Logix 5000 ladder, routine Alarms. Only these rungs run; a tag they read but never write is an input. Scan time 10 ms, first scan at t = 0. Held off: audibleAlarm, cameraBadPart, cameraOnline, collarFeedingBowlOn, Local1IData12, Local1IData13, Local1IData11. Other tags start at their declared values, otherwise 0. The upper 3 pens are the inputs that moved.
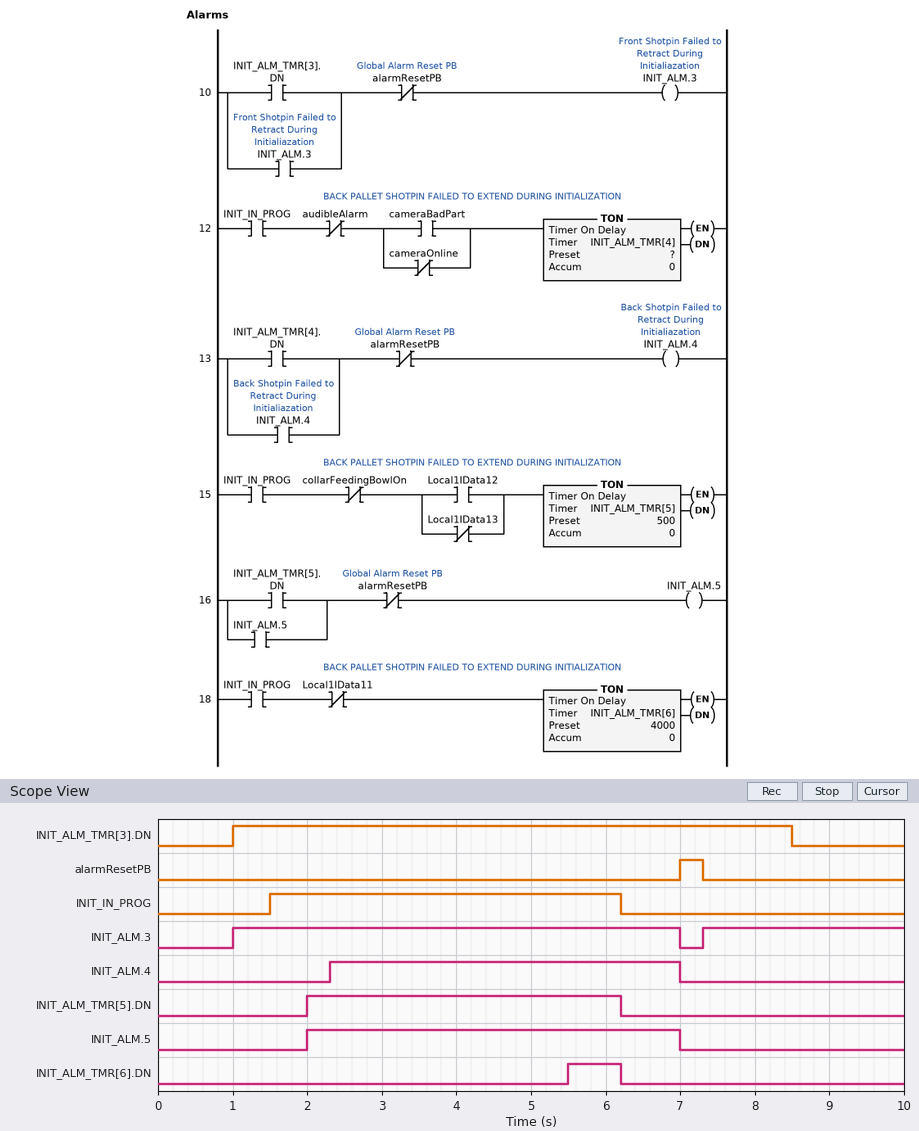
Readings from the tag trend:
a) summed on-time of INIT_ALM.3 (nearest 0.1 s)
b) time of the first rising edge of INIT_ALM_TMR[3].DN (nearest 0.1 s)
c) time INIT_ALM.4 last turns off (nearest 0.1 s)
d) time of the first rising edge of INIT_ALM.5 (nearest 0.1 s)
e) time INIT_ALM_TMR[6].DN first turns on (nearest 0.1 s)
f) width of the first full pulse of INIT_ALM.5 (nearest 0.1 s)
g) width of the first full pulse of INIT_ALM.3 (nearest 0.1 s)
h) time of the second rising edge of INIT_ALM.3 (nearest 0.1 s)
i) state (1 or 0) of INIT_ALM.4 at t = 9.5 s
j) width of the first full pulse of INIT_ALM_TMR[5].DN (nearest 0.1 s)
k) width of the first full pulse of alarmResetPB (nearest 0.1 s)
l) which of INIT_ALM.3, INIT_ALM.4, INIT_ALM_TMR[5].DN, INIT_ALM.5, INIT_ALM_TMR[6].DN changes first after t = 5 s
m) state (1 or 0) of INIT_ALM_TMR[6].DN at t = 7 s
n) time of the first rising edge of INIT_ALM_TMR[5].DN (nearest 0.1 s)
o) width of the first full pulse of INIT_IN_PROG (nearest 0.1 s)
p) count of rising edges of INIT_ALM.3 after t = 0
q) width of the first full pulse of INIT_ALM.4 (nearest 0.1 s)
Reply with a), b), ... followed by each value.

a) 8.7 s
b) 1.0 s
c) 7.0 s
d) 2.0 s
e) 5.5 s
f) 5.0 s
g) 6.0 s
h) 7.3 s
i) 0
j) 4.2 s
k) 0.3 s
l) INIT_ALM_TMR[6].DN
m) 0
n) 2.0 s
o) 4.7 s
p) 2
q) 4.7 s
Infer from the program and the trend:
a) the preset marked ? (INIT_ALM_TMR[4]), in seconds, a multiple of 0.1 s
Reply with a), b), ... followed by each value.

a) 0.8 s
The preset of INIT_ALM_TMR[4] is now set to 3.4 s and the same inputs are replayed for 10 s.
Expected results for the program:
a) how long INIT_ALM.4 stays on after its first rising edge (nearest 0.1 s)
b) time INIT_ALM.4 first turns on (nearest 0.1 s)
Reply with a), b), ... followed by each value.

a) 2.1 s
b) 4.9 s
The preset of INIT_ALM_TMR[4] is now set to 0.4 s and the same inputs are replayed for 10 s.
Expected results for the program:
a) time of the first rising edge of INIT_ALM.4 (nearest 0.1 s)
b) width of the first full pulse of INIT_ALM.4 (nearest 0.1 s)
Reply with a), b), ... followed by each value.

a) 1.9 s
b) 5.1 s
